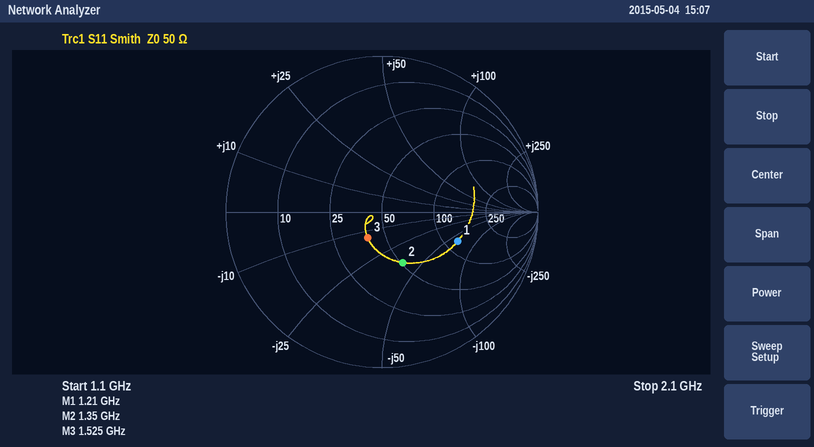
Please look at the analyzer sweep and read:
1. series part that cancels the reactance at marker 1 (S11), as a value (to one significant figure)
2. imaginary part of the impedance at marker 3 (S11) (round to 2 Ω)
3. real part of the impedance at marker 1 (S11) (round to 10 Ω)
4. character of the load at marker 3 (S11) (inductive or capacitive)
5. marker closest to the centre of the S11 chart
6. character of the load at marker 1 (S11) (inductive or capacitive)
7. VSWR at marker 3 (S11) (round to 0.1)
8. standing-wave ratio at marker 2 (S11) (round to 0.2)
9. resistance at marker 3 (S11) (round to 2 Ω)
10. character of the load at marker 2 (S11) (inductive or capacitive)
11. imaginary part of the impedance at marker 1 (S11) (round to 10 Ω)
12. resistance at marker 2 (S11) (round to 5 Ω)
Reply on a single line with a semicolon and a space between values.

8 nH; -14 Ω; 120 Ω; capacitive; marker 3; capacitive; 1.5; 2.0; 40 Ω; capacitive; -60 Ω; 50 Ω
